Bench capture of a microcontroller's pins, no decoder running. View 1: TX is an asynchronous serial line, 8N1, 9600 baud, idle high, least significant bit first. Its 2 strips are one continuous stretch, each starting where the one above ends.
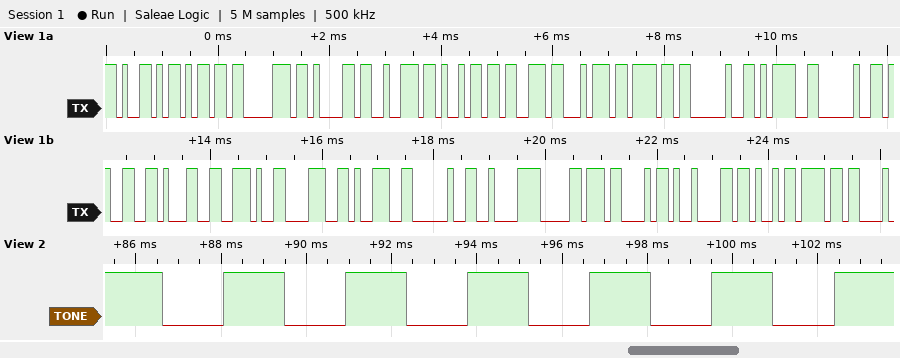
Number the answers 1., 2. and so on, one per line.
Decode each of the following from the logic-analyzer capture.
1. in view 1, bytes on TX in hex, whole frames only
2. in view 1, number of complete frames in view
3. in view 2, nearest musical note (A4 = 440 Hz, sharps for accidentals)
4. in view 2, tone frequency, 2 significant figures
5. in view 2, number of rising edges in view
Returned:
1. 59 6D 70 61 72 69 73 74 6F 20 3D 20 33 31 2E 38 39 20 C2 B0 43 09 4B 6F
2. 24
3. F4
4. 350 Hz
5. 6
